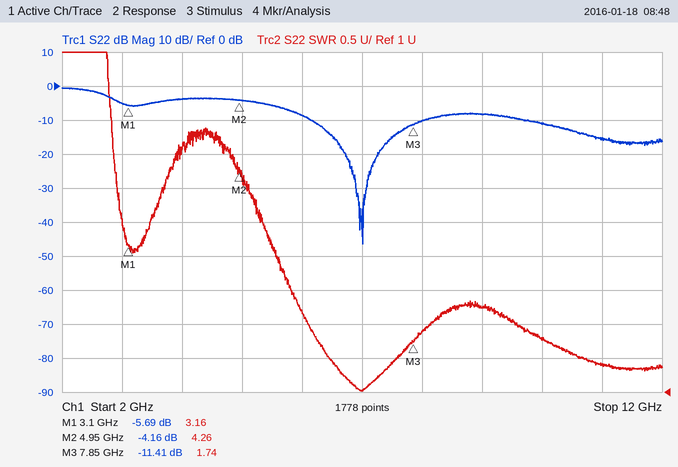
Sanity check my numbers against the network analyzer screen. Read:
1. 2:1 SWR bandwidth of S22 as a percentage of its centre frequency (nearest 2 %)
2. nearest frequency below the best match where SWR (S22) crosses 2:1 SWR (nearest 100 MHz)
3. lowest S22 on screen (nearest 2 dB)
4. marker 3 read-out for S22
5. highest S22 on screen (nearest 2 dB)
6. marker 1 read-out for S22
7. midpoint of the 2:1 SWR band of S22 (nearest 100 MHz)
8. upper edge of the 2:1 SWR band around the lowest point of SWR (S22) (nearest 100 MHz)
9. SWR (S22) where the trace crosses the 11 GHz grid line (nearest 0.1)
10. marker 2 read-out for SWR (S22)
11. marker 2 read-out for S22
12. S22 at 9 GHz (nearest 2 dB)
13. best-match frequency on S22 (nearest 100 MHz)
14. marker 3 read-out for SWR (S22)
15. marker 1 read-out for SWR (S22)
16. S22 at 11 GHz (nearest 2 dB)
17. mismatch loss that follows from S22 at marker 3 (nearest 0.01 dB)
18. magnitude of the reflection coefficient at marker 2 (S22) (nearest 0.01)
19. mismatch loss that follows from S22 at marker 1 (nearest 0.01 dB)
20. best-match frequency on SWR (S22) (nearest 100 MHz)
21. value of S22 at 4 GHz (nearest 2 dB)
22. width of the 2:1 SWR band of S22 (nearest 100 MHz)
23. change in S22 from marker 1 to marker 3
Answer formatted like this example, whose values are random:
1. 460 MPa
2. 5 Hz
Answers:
1. 28 %
2. 6.1 GHz
3. -46 dB
4. -11.41 dB
5. 0 dB
6. -5.69 dB
7. 7.1 GHz
8. 8.1 GHz
9. 1.4
10. 4.26
11. -4.16 dB
12. -8 dB
13. 7.0 GHz
14. 1.74
15. 3.16
16. -16 dB
17. 0.33 dB
18. 0.62
19. 1.37 dB
20. 7.0 GHz
21. -4 dB
22. 2.0 GHz
23. -5.72 dB
